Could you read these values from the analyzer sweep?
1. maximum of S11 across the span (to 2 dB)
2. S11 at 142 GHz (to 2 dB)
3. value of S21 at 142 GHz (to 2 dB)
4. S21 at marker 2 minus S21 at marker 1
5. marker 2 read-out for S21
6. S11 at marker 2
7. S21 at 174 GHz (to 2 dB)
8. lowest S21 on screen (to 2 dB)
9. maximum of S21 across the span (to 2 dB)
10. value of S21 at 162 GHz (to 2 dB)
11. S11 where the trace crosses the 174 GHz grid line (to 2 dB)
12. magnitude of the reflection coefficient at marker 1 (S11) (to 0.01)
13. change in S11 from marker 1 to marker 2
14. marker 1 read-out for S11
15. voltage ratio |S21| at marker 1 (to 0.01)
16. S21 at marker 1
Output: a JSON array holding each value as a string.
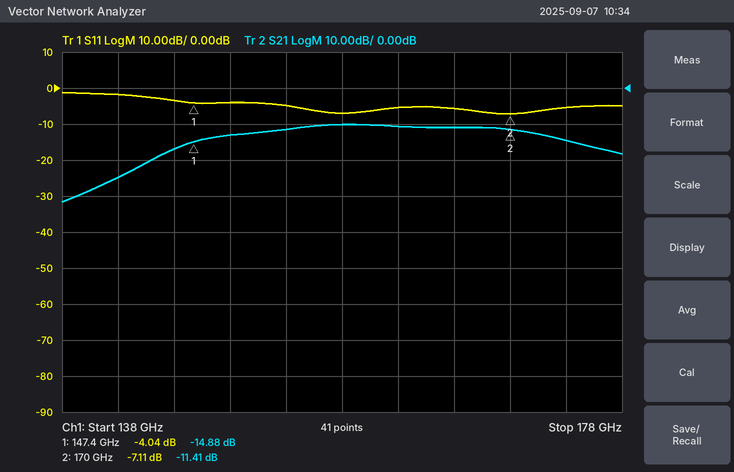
["-2 dB", "-2 dB", "-24 dB", "3.47 dB", "-11.41 dB", "-7.11 dB", "-14 dB", "-32 dB", "-10 dB", "-10 dB", "-6 dB", "0.63", "-3.07 dB", "-4.04 dB", "0.18", "-14.88 dB"]
